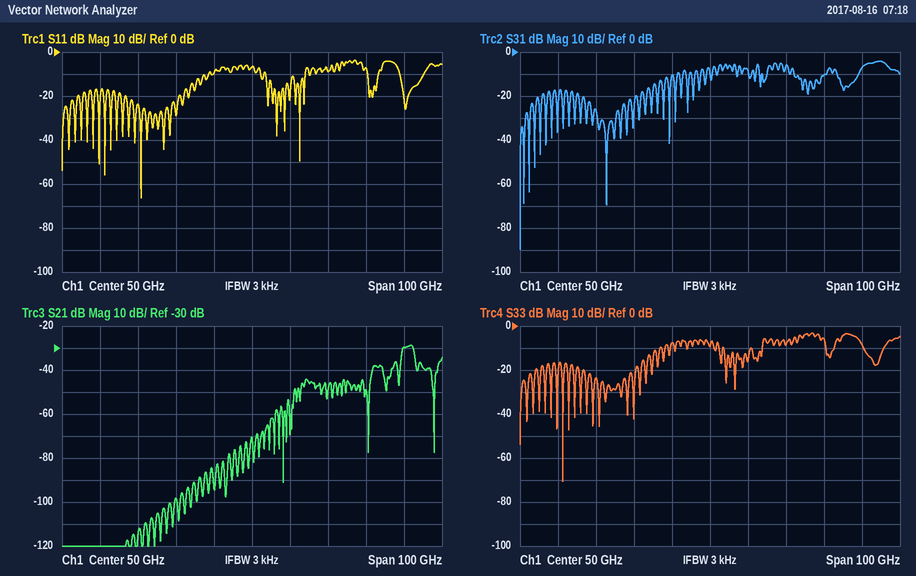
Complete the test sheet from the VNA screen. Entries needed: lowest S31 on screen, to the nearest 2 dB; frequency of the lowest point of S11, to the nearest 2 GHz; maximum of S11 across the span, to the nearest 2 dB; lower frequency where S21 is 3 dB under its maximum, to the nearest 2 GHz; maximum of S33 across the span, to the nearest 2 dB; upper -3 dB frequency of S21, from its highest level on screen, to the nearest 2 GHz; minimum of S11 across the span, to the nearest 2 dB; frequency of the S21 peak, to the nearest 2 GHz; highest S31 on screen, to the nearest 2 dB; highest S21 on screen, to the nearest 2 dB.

-90 dB
20 GHz
-4 dB
90 GHz
-4 dB
92 GHz
-66 dB
92 GHz
-4 dB
-28 dB
